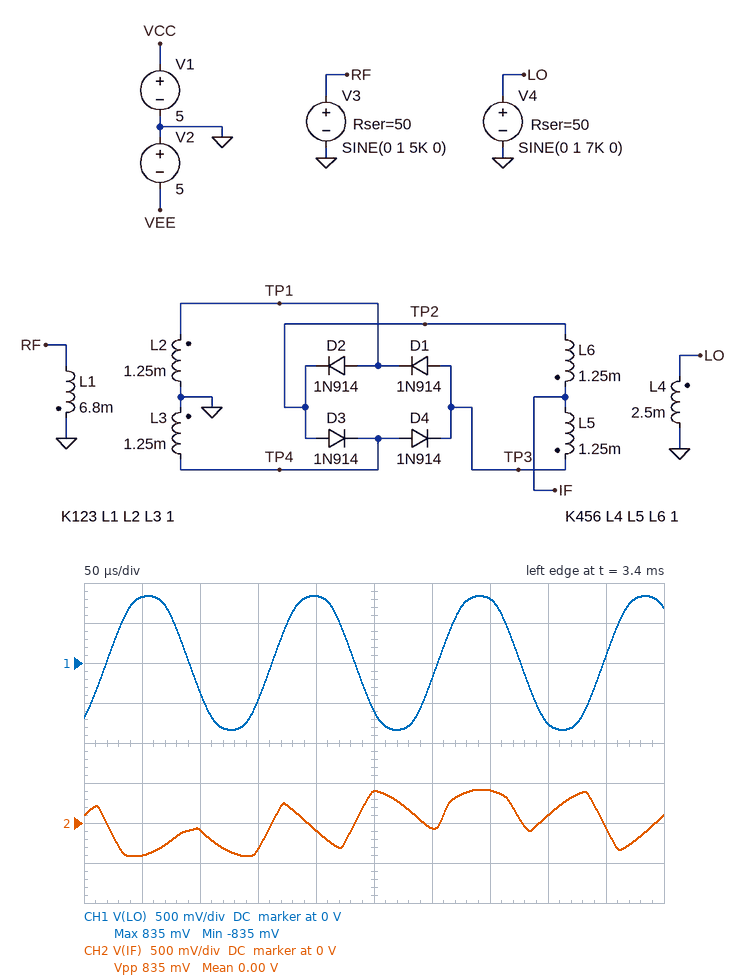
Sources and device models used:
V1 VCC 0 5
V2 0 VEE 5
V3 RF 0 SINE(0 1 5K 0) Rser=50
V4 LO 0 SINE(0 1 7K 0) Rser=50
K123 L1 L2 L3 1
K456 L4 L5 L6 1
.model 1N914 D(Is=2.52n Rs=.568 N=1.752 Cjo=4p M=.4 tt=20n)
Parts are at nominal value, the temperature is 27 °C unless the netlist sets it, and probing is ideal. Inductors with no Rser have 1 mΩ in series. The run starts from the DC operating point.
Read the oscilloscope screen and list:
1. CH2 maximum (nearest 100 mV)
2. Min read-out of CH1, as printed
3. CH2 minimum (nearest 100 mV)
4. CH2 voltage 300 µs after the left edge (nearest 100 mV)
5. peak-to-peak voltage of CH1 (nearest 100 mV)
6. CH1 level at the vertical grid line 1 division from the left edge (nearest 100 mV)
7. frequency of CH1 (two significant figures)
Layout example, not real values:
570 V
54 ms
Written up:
400 mV
-835 mV
-400 mV
-100 mV
1.7 V
800 mV
7.0 kHz
